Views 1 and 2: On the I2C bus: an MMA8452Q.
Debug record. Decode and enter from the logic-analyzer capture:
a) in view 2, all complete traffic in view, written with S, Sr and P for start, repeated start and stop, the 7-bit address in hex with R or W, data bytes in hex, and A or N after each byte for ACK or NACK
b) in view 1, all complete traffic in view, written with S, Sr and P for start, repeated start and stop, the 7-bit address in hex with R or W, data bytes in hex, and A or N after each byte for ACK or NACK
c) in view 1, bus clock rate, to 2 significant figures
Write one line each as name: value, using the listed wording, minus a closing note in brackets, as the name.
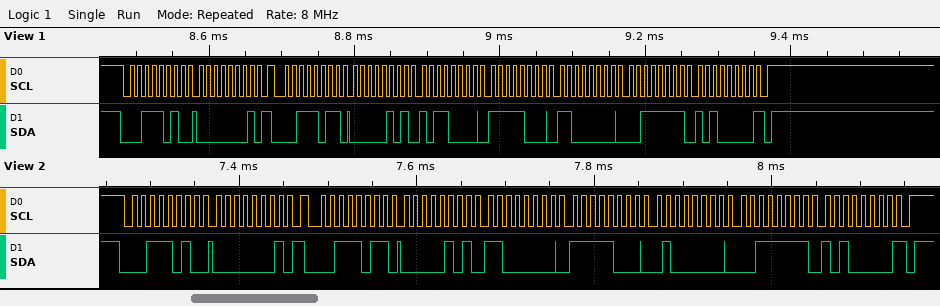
in view 2, all complete traffic in view, written with S, Sr and P for start, repeated start and stop, the 7-bit address in hex with R or W, data bytes in hex, and A or N after each byte for ACK or NACK: S 1DW A 01 A Sr 1DR A 05 A C0 A F8 A 40 A 3F A A0 N P
in view 1, all complete traffic in view, written with S, Sr and P for start, repeated start and stop, the 7-bit address in hex with R or W, data bytes in hex, and A or N after each byte for ACK or NACK: S 1DW A 01 A Sr 1DR A 05 A B0 A F8 A C0 A 3F A A0 N P
in view 1, bus clock rate, to 2 significant figures: 100 kHz
